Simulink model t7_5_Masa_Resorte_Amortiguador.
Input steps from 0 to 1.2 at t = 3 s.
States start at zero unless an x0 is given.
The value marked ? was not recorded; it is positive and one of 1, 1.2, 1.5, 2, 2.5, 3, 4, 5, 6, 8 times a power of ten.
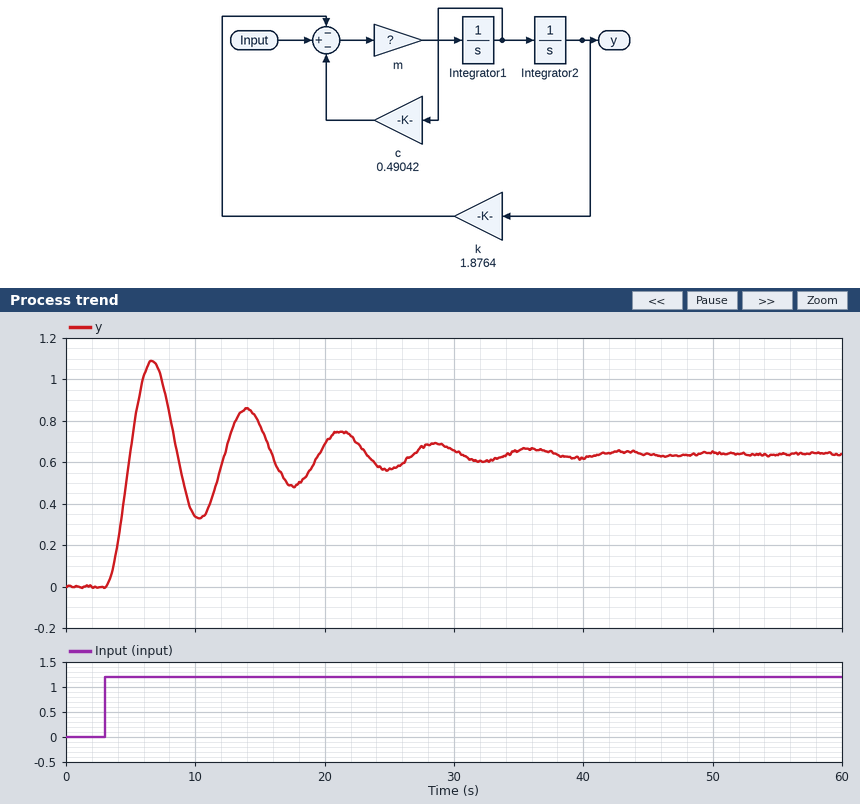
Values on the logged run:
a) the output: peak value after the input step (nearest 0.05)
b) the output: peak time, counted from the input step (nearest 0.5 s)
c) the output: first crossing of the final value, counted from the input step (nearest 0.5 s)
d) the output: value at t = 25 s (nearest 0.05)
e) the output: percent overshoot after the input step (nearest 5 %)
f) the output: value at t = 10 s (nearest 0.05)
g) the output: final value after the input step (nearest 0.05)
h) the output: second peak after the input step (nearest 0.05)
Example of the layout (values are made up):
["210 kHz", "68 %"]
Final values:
["1.10", "3.5 s", "2.0 s", "0.55", "70 %", "0.35", "0.65", "0.85"]
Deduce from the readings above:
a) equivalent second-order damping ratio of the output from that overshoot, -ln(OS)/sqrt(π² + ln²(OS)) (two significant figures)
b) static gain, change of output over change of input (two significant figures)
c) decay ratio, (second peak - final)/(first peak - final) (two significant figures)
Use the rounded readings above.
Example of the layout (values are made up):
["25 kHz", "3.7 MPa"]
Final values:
["0.11", "0.54", "0.44"]
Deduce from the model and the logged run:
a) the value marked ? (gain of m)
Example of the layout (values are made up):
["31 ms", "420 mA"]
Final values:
["0.4"]
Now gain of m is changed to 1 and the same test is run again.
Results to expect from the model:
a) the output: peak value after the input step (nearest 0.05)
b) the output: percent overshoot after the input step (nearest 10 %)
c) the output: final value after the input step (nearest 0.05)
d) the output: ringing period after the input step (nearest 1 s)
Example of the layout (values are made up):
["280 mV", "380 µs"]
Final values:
["1.00", "60 %", "0.65", "5 s"]
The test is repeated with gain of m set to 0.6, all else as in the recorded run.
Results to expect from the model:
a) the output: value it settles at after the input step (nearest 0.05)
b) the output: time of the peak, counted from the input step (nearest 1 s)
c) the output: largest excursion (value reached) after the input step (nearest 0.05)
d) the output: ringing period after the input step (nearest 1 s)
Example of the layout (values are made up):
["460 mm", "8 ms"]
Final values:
["0.65", "3 s", "1.05", "6 s"]
